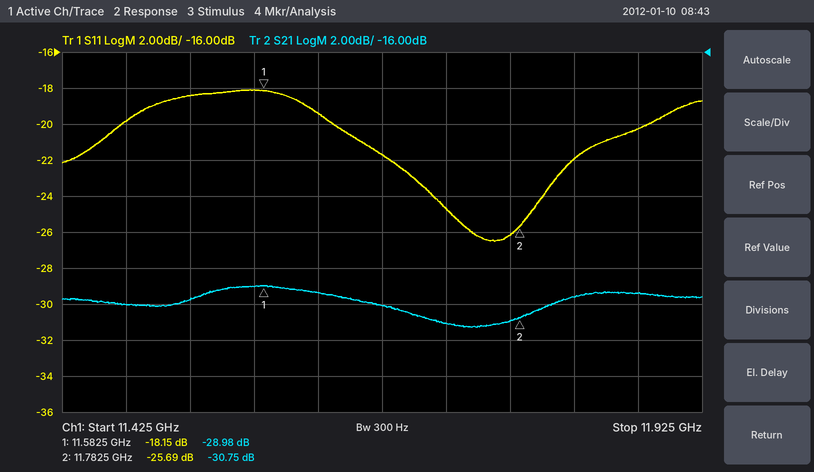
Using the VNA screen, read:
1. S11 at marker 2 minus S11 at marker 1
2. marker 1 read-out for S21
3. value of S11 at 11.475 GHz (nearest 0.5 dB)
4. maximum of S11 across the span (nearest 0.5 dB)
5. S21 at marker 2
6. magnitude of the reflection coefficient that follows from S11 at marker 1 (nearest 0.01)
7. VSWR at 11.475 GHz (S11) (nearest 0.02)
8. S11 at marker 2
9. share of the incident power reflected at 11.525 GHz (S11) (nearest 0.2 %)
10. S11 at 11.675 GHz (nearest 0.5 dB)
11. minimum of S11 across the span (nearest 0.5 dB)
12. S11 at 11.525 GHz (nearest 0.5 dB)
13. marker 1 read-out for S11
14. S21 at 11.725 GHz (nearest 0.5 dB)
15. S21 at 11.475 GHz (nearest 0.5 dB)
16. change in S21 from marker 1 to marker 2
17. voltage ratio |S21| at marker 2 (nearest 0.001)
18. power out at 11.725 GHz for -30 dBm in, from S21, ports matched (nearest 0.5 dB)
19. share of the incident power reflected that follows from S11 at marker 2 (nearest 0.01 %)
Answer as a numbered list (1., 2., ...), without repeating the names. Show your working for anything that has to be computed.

1. -25.69 − (-18.15) = -7.54 dB
2. -28.98 dB
3. -20.0 dB
4. -18.0 dB
5. -30.75 dB
6. 10^(-18.15/20) ≈ 0.12
7. |Γ| = 10^(-20/20) = 0.1000; VSWR = (1 + 0.1000)/(1 − 0.1000) ≈ 1.22
8. -25.69 dB
9. 10^(-18.5/10) ≈ 1.4 %
10. -21.5 dB
11. -26.5 dB
12. -18.5 dB
13. -18.15 dB
14. -31.0 dB
15. -30.0 dB
16. -30.75 − (-28.98) = -1.77 dB
17. 10^(-30.75/20) ≈ 0.029
18. -30 dBm + (-31.0 dB) = -61.0 dBm
19. 10^(-25.69/10) ≈ 0.27 %
